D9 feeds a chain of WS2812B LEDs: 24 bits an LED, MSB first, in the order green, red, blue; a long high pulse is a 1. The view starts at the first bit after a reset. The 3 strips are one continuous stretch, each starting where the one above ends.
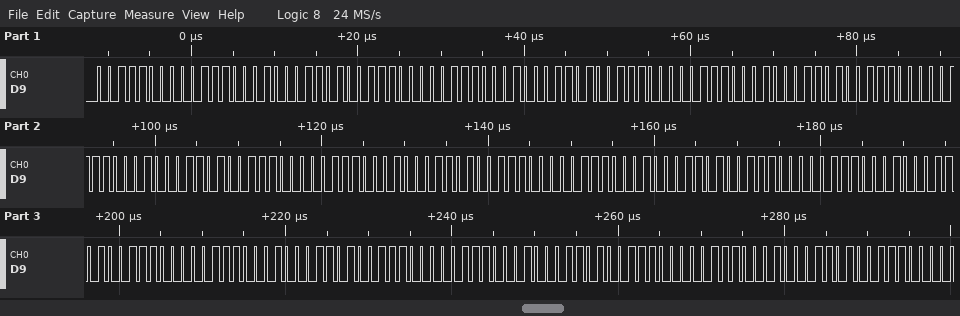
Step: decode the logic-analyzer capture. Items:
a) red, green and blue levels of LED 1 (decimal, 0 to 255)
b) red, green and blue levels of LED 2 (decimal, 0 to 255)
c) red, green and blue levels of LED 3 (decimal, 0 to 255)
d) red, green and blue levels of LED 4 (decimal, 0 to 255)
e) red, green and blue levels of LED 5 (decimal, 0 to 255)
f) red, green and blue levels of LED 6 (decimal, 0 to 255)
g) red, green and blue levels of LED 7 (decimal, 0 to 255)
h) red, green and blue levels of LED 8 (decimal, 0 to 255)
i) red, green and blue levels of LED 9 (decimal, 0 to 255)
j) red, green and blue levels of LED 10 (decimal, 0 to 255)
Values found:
56, 56, 141
56, 56, 141
56, 56, 141
56, 56, 141
56, 56, 141
56, 56, 141
56, 56, 141
56, 56, 141
56, 56, 141
56, 56, 141
